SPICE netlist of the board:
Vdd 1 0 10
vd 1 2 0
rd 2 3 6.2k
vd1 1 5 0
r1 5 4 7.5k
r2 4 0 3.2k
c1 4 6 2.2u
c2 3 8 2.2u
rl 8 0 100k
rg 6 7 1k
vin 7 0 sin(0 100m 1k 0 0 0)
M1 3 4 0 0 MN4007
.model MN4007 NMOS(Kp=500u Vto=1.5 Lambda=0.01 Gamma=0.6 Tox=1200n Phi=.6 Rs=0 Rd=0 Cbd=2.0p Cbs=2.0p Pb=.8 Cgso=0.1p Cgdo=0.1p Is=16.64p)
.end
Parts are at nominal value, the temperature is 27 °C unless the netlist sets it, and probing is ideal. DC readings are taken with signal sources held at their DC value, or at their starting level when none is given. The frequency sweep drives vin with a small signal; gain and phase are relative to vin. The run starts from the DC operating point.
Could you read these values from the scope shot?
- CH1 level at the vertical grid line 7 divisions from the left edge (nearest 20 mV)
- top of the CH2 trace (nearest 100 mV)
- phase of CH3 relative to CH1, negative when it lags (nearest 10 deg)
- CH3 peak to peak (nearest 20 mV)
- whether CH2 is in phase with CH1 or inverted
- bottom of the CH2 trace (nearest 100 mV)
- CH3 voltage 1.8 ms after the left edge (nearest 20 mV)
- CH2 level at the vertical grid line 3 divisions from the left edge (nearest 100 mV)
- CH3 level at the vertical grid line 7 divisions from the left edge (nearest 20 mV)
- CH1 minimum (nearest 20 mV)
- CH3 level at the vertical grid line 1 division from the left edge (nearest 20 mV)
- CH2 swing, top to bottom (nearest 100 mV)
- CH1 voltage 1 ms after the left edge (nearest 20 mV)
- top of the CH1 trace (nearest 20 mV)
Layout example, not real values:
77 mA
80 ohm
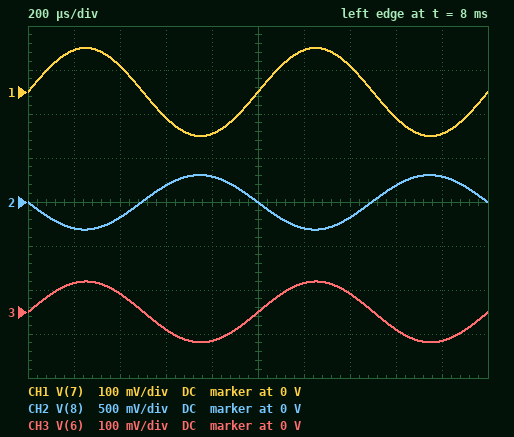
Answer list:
60 mV
300 mV
0 deg
140 mV
inverted
-300 mV
-60 mV
200 mV
40 mV
-100 mV
60 mV
600 mV
0 V
100 mV
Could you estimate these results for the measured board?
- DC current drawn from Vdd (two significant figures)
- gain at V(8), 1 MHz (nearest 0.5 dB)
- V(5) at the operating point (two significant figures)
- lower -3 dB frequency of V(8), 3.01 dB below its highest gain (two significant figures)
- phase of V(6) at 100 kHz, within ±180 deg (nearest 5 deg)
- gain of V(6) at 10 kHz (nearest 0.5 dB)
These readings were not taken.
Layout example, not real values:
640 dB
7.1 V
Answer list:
1.5 mA
10.0 dB
10 V
22 Hz
0 deg
-3.0 dB
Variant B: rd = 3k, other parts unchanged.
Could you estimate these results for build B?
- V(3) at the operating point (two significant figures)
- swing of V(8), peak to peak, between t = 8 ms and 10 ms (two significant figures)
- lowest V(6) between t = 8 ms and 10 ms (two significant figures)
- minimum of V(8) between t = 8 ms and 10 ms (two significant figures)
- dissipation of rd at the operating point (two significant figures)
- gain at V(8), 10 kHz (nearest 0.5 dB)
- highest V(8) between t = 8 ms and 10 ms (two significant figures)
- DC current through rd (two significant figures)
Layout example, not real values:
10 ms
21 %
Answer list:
8.2 V
320 mV
-69 mV
-160 mV
1.1 mW
4.0 dB
160 mV
600 µA
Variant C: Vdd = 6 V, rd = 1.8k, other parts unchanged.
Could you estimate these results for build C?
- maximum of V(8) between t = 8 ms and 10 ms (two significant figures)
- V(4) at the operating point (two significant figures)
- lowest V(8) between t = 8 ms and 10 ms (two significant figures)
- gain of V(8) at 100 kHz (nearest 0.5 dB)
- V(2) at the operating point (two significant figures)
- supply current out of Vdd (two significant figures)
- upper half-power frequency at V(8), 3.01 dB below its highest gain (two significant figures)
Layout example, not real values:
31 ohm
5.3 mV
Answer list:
17 mV
1.8 V
-21 mV
-14.5 dB
6.0 V
580 µA
130 MHz
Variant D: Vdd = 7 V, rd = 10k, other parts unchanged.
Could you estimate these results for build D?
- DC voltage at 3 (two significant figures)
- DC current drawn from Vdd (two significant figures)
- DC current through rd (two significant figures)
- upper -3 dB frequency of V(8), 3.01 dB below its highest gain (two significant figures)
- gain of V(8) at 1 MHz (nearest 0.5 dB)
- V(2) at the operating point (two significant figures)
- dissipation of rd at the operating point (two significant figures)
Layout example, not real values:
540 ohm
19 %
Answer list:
6.1 V
750 µA
93 µA
26 MHz
6.0 dB
7.0 V
87 µW
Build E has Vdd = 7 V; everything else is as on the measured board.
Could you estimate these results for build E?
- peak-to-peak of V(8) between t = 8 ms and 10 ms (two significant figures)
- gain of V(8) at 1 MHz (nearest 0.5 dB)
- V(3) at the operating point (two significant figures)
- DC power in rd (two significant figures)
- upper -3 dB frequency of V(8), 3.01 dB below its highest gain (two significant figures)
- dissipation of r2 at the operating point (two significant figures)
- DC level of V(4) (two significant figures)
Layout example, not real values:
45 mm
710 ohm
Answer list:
250 mV
2.0 dB
6.4 V
54 µW
41 MHz
1.4 mW
2.1 V
